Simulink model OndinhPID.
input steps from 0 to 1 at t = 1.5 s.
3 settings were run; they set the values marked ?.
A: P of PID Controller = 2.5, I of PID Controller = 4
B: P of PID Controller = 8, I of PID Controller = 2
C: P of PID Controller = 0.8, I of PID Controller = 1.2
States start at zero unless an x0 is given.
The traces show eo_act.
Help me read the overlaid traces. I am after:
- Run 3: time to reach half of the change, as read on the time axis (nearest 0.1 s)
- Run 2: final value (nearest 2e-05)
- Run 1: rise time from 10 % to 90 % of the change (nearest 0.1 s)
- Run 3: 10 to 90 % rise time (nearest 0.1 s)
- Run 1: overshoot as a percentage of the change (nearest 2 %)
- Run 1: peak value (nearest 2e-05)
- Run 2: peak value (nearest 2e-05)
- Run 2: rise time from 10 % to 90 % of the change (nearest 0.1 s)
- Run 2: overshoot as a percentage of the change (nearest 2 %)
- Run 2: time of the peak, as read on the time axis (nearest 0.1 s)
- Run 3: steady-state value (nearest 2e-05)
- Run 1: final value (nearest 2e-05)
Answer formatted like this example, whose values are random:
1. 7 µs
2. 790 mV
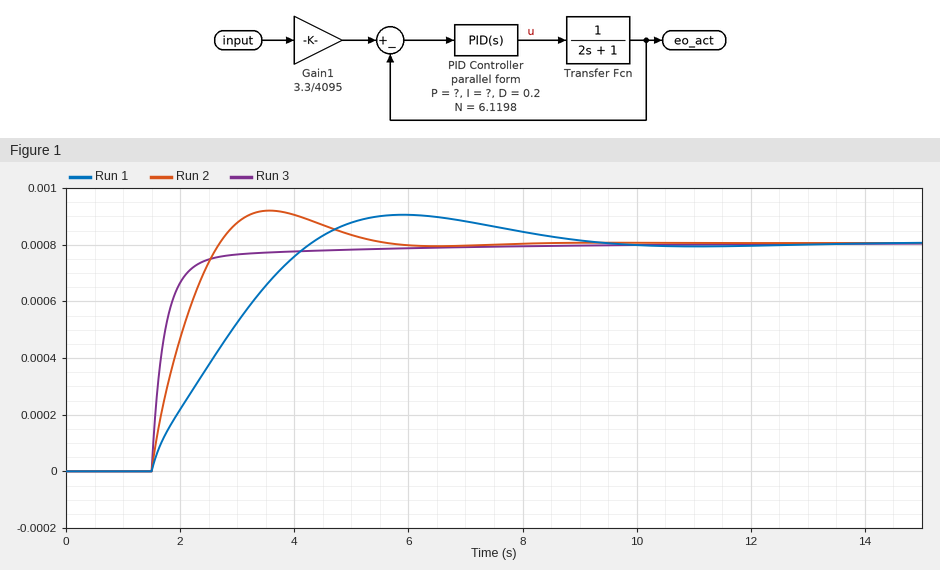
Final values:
1. 1.7 s
2. 0.00080
3. 2.2 s
4. 0.7 s
5. 12 %
6. 0.00090
7. 0.00092
8. 0.9 s
9. 14 %
10. 3.6 s
11. 0.00080
12. 0.00080
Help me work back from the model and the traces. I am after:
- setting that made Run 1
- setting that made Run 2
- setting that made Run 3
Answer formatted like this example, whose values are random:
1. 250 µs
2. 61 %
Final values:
1. C
2. A
3. B
